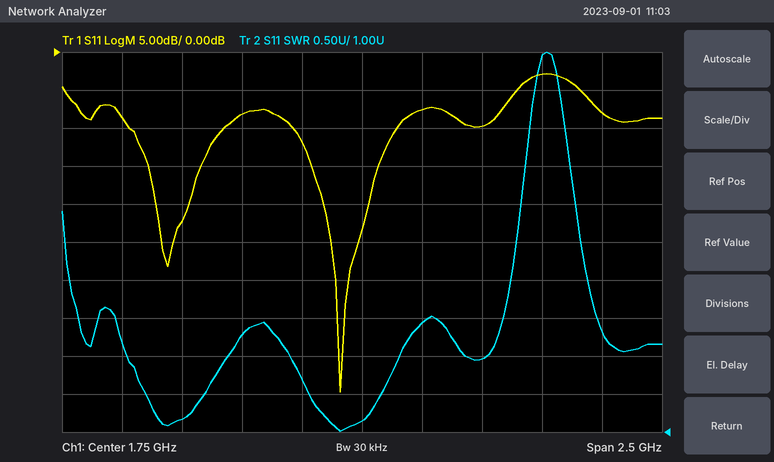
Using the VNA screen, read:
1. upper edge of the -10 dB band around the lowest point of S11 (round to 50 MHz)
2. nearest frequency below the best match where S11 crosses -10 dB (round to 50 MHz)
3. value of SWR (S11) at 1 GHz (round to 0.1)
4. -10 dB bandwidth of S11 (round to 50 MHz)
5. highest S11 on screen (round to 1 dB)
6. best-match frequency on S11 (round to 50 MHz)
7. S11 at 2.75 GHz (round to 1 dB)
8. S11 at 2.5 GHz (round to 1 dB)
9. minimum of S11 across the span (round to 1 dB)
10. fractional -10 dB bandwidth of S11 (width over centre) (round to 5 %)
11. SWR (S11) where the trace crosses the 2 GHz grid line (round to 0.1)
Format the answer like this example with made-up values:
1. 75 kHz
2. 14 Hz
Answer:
1. 1.90 GHz
2. 1.45 GHz
3. 1.2
4. 450 MHz
5. -3 dB
6. 1.65 GHz
7. -8 dB
8. -3 dB
9. -45 dB
10. 25 %
11. 2.4
